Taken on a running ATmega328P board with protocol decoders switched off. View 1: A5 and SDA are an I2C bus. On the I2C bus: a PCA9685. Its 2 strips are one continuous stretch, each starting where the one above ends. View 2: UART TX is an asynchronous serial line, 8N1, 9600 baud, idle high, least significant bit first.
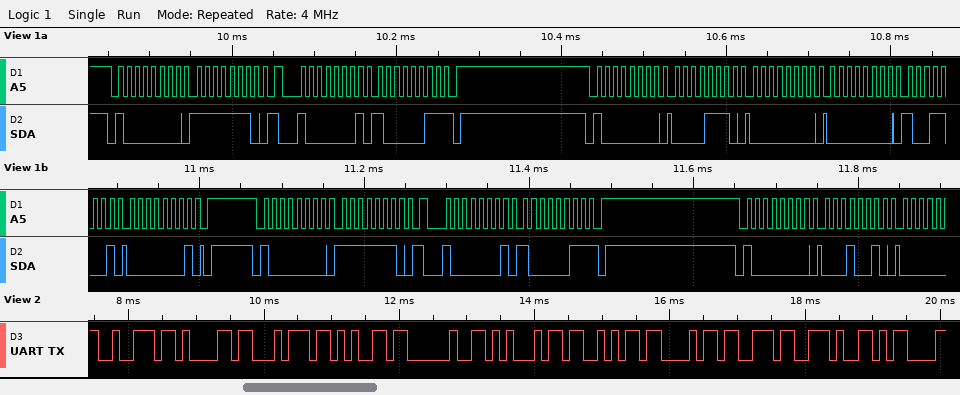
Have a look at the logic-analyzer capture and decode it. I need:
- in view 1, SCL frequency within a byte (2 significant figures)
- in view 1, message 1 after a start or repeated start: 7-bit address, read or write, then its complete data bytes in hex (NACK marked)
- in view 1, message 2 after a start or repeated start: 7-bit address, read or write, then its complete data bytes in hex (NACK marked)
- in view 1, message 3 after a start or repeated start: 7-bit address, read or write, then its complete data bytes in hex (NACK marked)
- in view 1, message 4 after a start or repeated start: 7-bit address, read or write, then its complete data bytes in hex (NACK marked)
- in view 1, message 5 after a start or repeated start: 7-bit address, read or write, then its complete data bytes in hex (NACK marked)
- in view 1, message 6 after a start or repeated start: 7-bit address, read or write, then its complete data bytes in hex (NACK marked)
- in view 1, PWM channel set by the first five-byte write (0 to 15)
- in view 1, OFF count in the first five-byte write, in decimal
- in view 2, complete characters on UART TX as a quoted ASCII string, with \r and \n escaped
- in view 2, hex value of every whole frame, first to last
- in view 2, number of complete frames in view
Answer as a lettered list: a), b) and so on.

a) 100 kHz
b) 0x40 write: FE
c) 0x40 read: 83 NACK
d) 0x40 write: 0E 00 00 99 01
e) 0x40 write: FE
f) 0x40 read: 83 NACK
g) 0x40 write: 12
h) 2
i) 409
j) "rate ESCs.\r"
k) 72 61 74 65 20 45 53 43 73 2E 0D
l) 11
